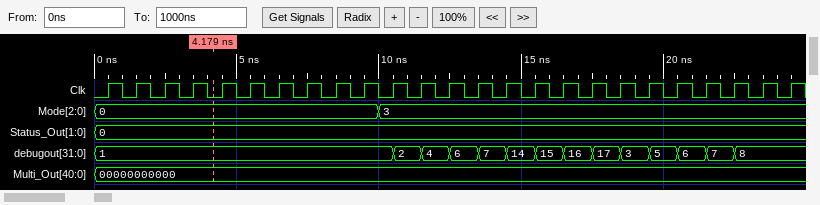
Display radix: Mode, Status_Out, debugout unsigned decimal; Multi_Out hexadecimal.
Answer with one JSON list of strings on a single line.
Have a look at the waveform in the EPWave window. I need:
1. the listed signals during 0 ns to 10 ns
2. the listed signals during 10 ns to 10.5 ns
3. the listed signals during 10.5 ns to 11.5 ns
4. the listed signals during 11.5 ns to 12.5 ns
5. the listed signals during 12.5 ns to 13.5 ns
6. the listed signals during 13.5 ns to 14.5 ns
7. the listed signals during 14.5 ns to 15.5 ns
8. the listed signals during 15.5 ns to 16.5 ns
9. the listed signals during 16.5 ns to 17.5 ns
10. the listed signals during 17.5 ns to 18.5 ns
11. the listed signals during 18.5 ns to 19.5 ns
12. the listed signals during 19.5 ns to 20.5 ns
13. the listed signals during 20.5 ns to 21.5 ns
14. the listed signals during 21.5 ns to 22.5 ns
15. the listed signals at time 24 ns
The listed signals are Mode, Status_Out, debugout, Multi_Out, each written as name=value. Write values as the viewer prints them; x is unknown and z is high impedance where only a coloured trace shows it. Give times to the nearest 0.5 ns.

["Mode=0, Status_Out=0, debugout=1, Multi_Out=00000000000", "Mode=3, Status_Out=0, debugout=1, Multi_Out=00000000000", "Mode=3, Status_Out=0, debugout=2, Multi_Out=00000000000", "Mode=3, Status_Out=0, debugout=4, Multi_Out=00000000000", "Mode=3, Status_Out=0, debugout=6, Multi_Out=00000000000", "Mode=3, Status_Out=0, debugout=7, Multi_Out=00000000000", "Mode=3, Status_Out=0, debugout=14, Multi_Out=00000000000", "Mode=3, Status_Out=0, debugout=15, Multi_Out=00000000000", "Mode=3, Status_Out=0, debugout=16, Multi_Out=00000000000", "Mode=3, Status_Out=0, debugout=17, Multi_Out=00000000000", "Mode=3, Status_Out=0, debugout=3, Multi_Out=00000000000", "Mode=3, Status_Out=0, debugout=5, Multi_Out=00000000000", "Mode=3, Status_Out=0, debugout=6, Multi_Out=00000000000", "Mode=3, Status_Out=0, debugout=7, Multi_Out=00000000000", "Mode=3, Status_Out=0, debugout=8, Multi_Out=00000000000"]
